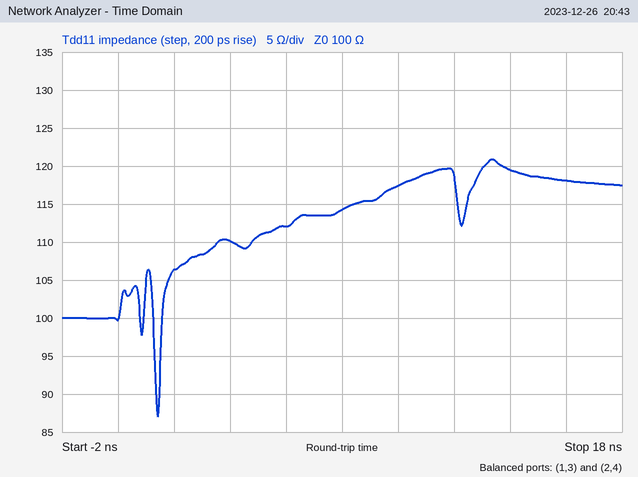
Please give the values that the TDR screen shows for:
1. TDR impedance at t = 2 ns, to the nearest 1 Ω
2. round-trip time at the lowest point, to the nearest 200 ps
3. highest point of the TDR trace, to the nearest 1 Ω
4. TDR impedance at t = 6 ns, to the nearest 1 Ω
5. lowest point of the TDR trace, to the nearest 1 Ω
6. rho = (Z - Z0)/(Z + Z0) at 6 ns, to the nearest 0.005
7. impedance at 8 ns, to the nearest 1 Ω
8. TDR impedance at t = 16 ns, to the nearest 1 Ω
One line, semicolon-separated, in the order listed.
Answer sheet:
106 Ω; 1.4 ns; 121 Ω; 112 Ω; 87 Ω; +0.055; 114 Ω; 118 Ω
